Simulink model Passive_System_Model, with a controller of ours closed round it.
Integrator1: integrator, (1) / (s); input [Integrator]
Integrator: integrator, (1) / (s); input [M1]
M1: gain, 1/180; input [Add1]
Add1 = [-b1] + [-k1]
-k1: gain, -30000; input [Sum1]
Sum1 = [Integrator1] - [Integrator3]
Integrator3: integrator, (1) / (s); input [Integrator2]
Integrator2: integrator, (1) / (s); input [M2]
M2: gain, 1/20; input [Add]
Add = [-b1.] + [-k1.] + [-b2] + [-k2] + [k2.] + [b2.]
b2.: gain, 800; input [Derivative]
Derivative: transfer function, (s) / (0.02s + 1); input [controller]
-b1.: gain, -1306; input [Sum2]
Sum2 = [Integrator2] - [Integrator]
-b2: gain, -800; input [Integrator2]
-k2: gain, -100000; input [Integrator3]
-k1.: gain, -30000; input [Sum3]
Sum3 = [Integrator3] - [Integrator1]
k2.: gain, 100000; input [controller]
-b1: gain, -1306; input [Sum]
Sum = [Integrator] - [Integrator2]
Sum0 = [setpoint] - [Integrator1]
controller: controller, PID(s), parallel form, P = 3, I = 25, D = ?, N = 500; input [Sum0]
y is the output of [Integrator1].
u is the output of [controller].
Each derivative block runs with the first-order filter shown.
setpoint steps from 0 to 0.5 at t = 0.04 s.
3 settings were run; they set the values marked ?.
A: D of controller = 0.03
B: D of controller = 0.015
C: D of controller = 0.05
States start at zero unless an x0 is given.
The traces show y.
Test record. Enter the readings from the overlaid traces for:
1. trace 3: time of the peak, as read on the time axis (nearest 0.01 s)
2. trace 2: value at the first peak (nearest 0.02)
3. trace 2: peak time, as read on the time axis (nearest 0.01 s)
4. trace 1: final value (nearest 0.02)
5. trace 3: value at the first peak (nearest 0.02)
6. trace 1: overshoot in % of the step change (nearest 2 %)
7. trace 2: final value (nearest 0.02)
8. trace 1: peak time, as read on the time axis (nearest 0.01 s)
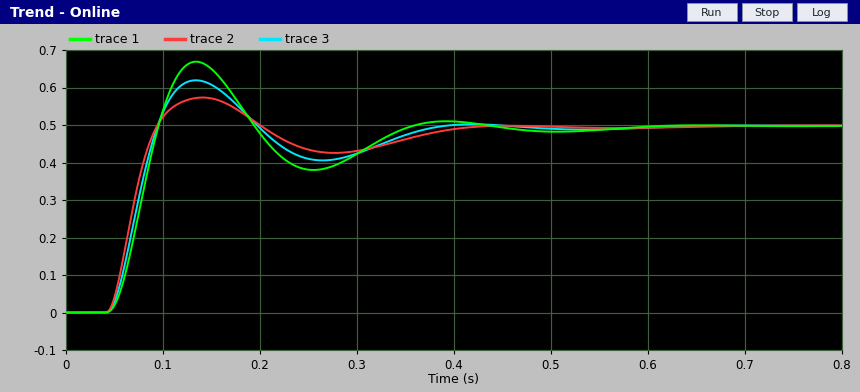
0.13 s
0.58
0.14 s
0.50
0.62
34 %
0.50
0.13 s
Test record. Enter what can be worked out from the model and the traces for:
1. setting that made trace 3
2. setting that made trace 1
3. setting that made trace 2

A
B
C
